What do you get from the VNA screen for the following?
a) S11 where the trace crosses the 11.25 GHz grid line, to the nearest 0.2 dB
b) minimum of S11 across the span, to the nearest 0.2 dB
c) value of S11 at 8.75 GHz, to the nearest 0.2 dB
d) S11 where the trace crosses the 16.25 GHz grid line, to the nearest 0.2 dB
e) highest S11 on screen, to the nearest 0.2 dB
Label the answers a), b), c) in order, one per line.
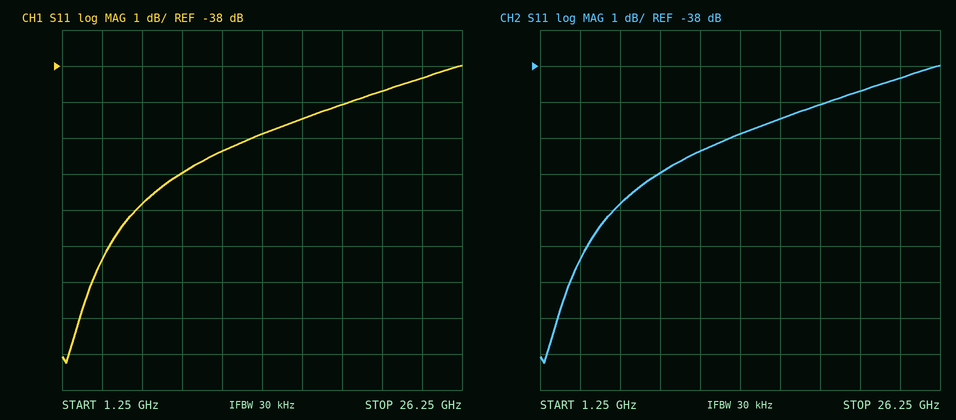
a) -40.4 dB
b) -46.2 dB
c) -41.0 dB
d) -39.4 dB
e) -38.0 dB
